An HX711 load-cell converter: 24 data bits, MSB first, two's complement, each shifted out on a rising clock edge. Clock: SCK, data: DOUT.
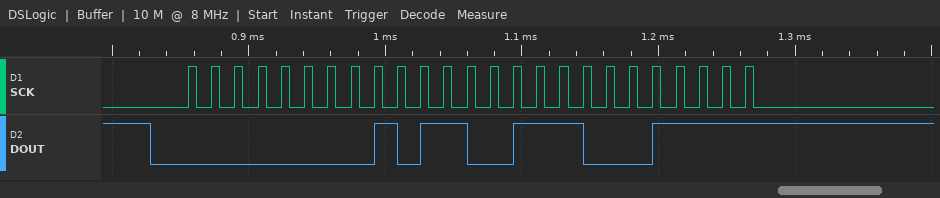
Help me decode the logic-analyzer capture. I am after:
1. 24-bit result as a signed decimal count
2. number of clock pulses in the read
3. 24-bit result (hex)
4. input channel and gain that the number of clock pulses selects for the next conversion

45967
25
0x00B38F
channel A, gain 128
